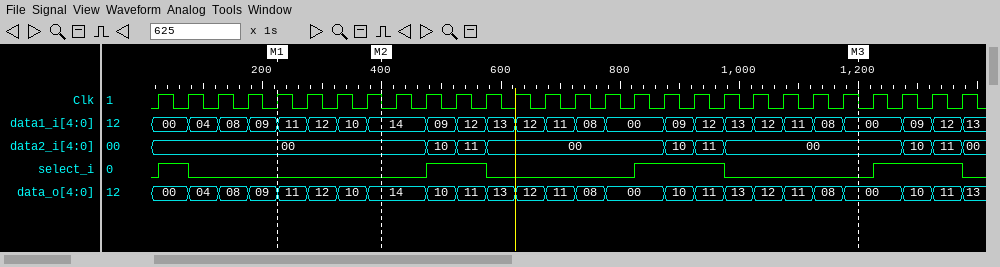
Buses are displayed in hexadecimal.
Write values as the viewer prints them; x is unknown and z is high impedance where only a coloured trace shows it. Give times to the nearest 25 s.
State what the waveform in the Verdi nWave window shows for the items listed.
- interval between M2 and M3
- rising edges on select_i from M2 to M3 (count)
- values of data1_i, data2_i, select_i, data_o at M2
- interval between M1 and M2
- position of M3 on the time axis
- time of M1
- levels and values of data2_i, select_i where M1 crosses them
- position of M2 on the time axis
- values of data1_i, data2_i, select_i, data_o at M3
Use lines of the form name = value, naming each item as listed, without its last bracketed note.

interval between M2 and M3 = 800 s
rising edges on select_i from M2 to M3 = 2
values of data1_i, data2_i, select_i, data_o at M2 = data1_i=14, data2_i=00, select_i=0, data_o=14
interval between M1 and M2 = 175 s
position of M3 on the time axis = 1200 s
time of M1 = 225 s
levels and values of data2_i, select_i where M1 crosses them = data2_i=00, select_i=0
position of M2 on the time axis = 400 s
values of data1_i, data2_i, select_i, data_o at M3 = data1_i=00, data2_i=00, select_i=0, data_o=00
